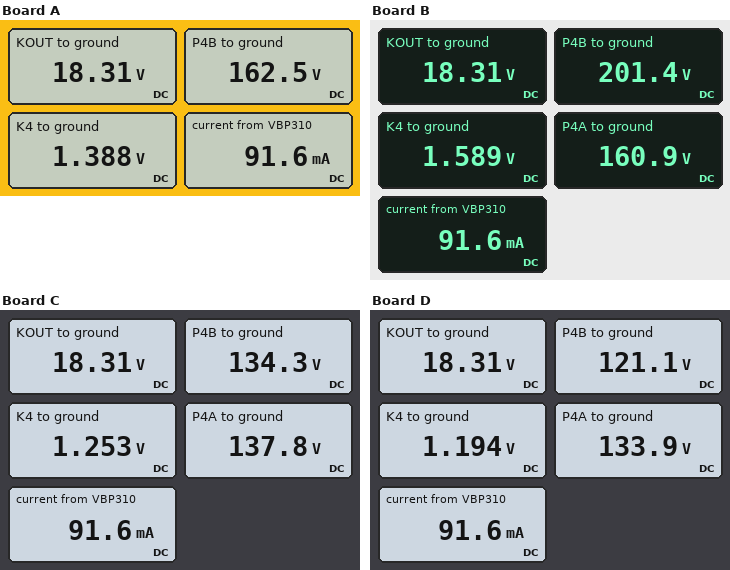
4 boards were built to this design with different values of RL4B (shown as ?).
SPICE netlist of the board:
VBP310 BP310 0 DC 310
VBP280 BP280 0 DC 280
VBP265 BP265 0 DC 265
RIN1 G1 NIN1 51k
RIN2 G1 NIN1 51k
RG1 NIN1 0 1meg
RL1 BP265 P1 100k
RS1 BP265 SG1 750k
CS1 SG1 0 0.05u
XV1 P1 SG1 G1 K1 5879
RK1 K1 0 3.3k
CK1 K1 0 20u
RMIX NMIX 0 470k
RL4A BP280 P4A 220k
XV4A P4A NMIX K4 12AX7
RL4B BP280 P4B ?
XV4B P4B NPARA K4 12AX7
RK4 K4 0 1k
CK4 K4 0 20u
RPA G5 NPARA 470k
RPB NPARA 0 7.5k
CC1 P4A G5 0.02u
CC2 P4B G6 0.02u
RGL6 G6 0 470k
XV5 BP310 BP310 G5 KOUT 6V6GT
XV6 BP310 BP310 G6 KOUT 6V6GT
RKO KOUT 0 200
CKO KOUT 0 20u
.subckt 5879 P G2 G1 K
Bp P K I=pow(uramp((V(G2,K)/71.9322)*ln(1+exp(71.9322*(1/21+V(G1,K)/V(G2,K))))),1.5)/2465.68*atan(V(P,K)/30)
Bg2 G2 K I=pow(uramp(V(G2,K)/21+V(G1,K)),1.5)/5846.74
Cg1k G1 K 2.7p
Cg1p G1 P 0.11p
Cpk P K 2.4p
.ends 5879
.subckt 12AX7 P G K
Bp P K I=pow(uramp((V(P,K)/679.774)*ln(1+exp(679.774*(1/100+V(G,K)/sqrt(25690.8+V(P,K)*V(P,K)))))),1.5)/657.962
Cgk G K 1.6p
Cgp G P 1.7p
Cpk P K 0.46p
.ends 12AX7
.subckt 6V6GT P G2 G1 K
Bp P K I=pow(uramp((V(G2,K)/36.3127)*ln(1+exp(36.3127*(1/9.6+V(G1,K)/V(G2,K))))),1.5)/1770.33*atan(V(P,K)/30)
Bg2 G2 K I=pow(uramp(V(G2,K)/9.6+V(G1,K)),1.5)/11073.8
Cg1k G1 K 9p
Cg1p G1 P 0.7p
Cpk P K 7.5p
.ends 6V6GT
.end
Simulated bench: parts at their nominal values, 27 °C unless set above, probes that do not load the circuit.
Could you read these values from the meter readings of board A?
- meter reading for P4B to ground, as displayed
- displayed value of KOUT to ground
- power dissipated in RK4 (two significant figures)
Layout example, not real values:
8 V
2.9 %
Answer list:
162.5 V
18.31 V
1.9 mW
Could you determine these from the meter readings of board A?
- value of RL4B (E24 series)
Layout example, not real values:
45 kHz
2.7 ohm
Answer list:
150 kΩ
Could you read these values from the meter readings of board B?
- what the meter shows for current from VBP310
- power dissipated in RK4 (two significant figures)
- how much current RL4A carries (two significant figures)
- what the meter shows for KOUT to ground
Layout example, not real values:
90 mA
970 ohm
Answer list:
91.6 mA
2.5 mW
540 µA
18.31 V
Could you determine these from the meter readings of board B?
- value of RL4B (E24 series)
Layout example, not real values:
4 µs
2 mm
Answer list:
75 kΩ
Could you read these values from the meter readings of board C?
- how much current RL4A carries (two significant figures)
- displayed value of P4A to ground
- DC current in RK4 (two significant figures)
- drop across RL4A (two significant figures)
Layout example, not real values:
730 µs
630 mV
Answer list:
650 µA
137.8 V
1.3 mA
140 V
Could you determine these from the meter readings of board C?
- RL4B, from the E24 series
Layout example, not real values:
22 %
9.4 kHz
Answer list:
240 kΩ
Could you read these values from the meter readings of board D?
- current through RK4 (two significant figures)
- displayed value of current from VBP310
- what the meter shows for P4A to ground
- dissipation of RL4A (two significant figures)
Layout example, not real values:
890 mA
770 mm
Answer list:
1.2 mA
91.6 mA
133.9 V
97 mW
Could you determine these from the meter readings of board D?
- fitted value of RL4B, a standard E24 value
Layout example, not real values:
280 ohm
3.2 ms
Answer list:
300 kΩ
